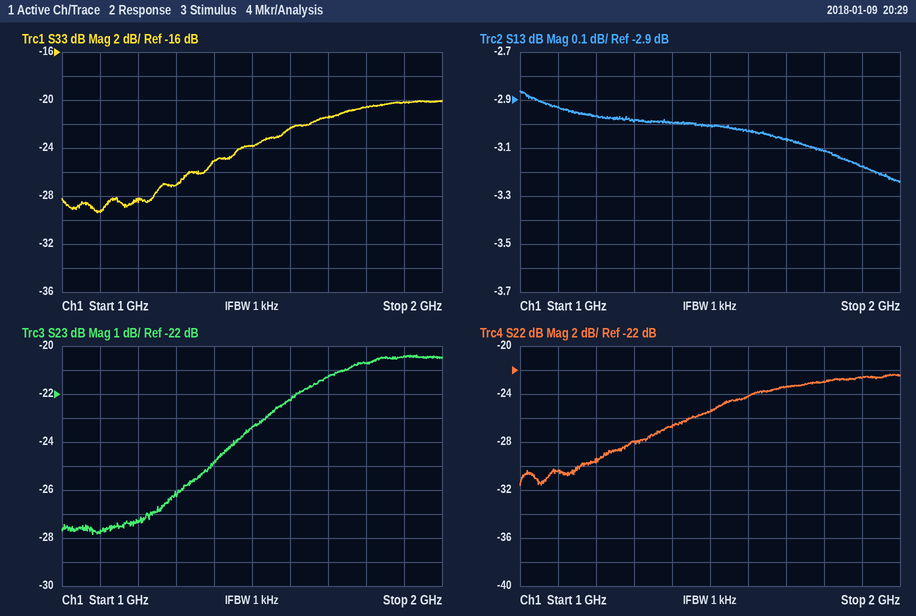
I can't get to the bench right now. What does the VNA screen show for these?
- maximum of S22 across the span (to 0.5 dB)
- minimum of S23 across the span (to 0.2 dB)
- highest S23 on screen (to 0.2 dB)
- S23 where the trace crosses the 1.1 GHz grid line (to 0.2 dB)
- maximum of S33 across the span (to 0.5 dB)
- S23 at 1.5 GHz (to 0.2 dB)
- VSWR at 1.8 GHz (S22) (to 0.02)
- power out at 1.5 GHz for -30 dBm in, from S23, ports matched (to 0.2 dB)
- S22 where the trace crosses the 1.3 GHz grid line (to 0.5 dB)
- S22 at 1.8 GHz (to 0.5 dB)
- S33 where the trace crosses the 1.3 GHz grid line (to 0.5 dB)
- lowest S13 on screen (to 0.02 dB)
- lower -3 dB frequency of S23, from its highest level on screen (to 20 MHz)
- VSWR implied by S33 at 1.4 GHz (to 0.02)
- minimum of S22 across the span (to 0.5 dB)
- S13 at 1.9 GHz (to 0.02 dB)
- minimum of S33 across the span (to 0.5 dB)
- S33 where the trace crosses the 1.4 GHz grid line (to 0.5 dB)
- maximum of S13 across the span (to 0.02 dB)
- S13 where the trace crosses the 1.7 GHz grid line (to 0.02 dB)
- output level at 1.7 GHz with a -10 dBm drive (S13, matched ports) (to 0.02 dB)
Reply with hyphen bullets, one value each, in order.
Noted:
- -22.5 dB
- -27.8 dB
- -20.4 dB
- -27.8 dB
- -20.0 dB
- -23.4 dB
- 1.16
- -53.4 dBm
- -28.0 dB
- -23.0 dB
- -27.0 dB
- -3.24 dB
- 1.50 GHz
- 1.12
- -31.5 dB
- -3.18 dB
- -29.5 dB
- -25.0 dB
- -2.86 dB
- -3.06 dB
- -13.06 dBm
